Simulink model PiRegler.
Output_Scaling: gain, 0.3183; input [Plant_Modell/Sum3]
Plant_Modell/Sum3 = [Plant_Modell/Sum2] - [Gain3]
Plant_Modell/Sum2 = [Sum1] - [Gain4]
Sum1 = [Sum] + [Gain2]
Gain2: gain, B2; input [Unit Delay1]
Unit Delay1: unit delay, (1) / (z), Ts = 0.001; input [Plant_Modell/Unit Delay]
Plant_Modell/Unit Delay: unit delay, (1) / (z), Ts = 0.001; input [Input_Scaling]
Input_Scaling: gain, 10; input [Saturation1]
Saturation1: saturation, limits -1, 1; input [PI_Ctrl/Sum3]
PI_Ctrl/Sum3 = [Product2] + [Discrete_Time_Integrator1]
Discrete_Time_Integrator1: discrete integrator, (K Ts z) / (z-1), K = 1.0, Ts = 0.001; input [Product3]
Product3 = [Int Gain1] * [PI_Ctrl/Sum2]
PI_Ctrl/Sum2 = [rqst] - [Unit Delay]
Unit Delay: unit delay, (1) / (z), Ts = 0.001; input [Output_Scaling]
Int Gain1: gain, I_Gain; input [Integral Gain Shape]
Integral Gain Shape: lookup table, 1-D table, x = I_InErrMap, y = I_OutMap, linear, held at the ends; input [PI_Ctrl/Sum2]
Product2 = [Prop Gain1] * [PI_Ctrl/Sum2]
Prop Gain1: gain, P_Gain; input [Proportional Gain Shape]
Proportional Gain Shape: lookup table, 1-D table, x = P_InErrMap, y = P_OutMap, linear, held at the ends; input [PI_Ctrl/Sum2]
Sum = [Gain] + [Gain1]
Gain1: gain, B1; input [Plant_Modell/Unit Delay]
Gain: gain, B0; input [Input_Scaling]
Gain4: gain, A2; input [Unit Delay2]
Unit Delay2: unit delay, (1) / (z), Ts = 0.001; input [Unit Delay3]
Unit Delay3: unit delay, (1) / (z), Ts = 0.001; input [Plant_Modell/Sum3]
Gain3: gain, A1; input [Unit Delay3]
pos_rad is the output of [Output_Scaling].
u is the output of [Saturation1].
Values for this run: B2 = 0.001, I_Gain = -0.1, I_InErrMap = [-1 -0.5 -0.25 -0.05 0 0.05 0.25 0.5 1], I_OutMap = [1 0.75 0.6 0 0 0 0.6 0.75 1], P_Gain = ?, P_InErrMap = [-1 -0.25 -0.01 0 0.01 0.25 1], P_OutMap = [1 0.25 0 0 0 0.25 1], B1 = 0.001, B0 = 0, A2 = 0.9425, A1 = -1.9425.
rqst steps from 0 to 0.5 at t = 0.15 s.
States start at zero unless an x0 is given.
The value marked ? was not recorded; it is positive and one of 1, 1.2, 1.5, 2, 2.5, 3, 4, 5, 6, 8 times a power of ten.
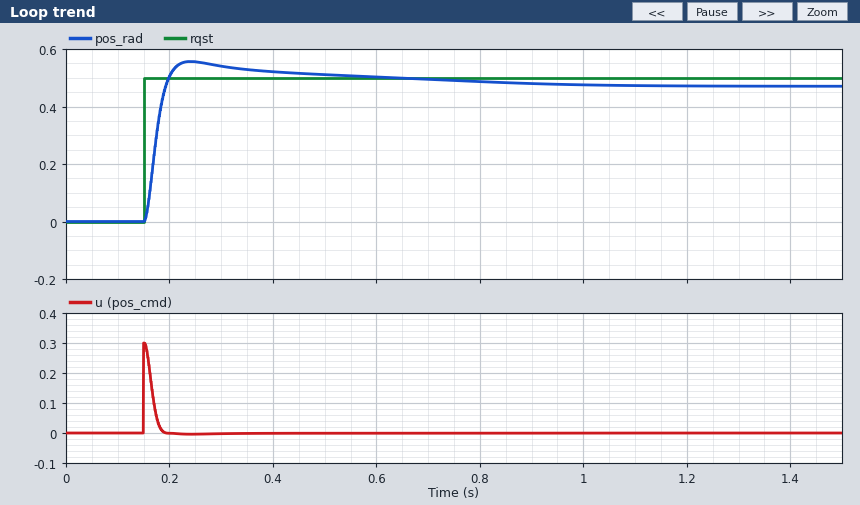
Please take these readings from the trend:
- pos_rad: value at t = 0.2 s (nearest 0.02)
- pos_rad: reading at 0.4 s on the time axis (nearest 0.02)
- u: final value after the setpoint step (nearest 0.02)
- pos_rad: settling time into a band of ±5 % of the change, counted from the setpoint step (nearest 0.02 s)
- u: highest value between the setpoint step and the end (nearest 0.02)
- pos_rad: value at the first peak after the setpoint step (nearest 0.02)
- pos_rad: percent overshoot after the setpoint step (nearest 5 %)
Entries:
0.50
0.52
0.00
0.56 s
0.30
0.56
20 %
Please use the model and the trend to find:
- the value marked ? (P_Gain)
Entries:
1.2
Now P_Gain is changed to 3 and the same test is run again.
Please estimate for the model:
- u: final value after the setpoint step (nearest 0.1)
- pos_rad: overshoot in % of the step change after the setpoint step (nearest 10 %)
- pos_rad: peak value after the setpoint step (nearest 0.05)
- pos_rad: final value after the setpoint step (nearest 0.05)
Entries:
0.0
50 %
0.70
0.50
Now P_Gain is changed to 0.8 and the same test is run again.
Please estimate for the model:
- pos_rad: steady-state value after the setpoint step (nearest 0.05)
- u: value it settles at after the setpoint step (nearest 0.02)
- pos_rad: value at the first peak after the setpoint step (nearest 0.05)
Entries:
0.45
0.00
0.50
